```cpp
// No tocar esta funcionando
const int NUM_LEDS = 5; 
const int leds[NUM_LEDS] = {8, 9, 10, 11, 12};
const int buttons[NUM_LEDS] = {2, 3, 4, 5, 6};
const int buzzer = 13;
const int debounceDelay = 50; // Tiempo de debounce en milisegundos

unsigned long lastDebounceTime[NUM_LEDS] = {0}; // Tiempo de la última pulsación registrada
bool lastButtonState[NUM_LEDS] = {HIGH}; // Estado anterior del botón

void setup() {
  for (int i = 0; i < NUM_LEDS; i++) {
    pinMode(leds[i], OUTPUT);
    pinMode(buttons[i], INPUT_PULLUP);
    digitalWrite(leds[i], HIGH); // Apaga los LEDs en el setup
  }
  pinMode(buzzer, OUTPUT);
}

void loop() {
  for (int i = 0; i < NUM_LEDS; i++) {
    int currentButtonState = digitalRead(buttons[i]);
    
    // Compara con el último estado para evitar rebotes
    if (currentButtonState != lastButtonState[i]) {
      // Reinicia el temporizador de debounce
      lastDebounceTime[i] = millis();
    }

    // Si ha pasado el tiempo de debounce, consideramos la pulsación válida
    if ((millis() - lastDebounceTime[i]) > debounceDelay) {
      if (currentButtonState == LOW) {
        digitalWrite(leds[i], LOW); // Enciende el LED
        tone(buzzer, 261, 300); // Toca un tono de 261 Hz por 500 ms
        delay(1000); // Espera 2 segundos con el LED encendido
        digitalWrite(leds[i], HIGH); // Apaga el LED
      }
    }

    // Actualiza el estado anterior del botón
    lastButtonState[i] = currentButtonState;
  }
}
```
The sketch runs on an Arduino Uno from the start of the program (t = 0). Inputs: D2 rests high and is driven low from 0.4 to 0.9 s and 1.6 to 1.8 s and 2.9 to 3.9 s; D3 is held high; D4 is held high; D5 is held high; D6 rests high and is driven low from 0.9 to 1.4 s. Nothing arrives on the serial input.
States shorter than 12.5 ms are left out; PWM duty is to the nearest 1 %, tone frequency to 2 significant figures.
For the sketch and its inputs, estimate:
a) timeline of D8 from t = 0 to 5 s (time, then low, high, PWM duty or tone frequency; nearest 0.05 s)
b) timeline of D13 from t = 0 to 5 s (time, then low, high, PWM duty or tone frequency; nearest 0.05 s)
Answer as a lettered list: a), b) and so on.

a) 0 s high; 0.45 s low; 1.45 s high; 1.65 s low; 2.65 s high; 2.95 s low; 3.95 s high
b) 0 s low; 0.45 s tone 260 Hz; 0.75 s low; 1.65 s tone 260 Hz; 1.95 s low; 2.95 s tone 260 Hz; 3.25 s low
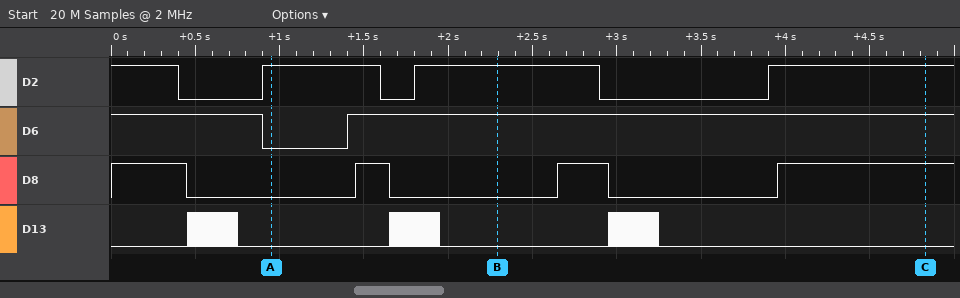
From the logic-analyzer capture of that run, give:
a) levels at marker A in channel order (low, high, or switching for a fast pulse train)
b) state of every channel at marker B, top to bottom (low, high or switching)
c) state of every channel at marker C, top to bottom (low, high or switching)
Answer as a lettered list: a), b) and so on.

a) D2 high, D6 low, D8 low, D13 low
b) D2 high, D6 high, D8 low, D13 low
c) D2 high, D6 high, D8 high, D13 low
